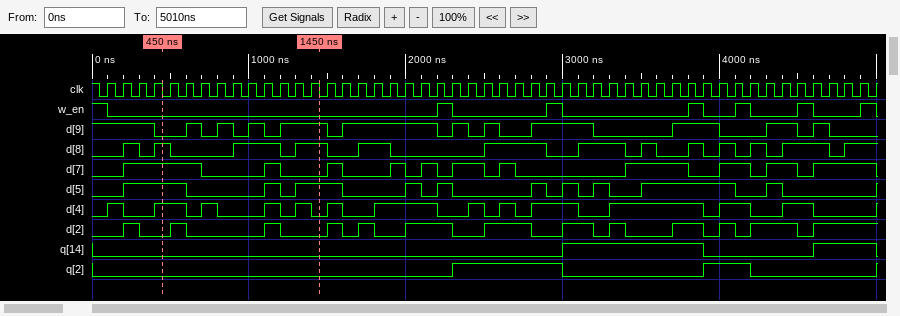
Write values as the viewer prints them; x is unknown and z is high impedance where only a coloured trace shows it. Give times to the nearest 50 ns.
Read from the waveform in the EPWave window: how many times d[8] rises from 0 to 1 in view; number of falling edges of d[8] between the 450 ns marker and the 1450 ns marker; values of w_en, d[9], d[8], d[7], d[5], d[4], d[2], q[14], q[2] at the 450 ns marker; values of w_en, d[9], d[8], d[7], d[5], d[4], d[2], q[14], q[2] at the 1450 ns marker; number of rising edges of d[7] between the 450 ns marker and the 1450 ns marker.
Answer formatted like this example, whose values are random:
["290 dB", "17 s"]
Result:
["13", "2", "w_en=0, d[9]=0, d[8]=1, d[7]=1, d[5]=1, d[4]=1, d[2]=0, q[14]=0, q[2]=0", "w_en=0, d[9]=1, d[8]=1, d[7]=0, d[5]=1, d[4]=0, d[2]=0, q[14]=0, q[2]=0", "1"]
